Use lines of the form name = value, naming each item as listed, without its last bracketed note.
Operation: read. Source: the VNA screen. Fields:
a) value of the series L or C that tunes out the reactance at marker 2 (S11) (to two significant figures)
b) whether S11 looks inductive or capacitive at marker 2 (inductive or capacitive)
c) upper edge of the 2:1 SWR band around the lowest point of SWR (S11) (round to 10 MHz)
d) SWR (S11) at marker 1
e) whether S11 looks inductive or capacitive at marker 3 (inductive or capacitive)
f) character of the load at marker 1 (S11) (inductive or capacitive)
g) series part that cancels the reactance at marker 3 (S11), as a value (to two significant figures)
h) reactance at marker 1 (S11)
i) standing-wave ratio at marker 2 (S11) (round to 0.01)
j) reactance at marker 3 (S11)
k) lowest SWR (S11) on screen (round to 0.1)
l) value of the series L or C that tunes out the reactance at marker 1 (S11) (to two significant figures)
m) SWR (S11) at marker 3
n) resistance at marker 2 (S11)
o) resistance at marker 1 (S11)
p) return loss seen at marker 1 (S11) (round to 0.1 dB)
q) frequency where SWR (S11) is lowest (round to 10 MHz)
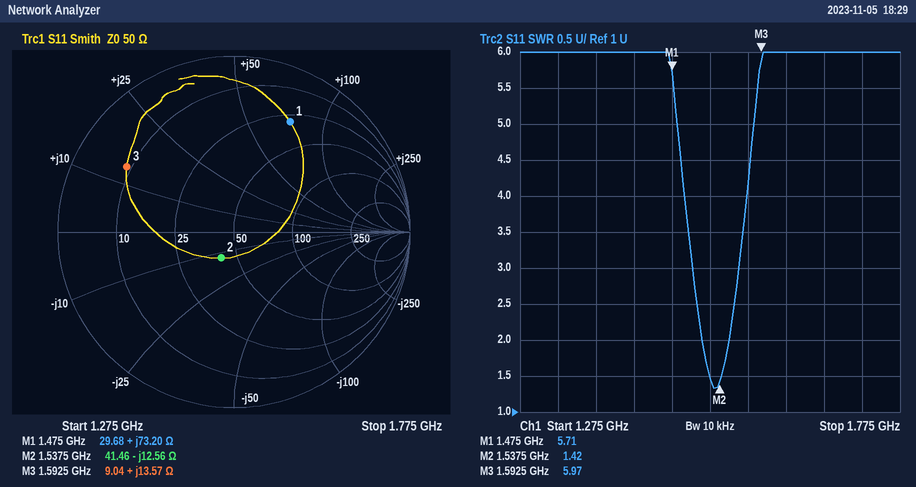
value of the series L or C that tunes out the reactance at marker 2 (S11) = 1.3 nH
whether S11 looks inductive or capacitive at marker 2 = capacitive
upper edge of the 2:1 SWR band around the lowest point of SWR (S11) = 1.55 GHz
SWR (S11) at marker 1 = 5.71
whether S11 looks inductive or capacitive at marker 3 = inductive
character of the load at marker 1 (S11) = inductive
series part that cancels the reactance at marker 3 (S11), as a value = 7.4 pF
reactance at marker 1 = +73.20 Ω
standing-wave ratio at marker 2 (S11) = 1.39
reactance at marker 3 = +13.57 Ω
lowest SWR (S11) on screen = 1.3
value of the series L or C that tunes out the reactance at marker 1 (S11) = 1.5 pF
SWR (S11) at marker 3 = 5.97
resistance at marker 2 = 41.46 Ω
resistance at marker 1 = 29.68 Ω
return loss seen at marker 1 (S11) = 3.1 dB
frequency where SWR (S11) is lowest = 1.53 GHz
